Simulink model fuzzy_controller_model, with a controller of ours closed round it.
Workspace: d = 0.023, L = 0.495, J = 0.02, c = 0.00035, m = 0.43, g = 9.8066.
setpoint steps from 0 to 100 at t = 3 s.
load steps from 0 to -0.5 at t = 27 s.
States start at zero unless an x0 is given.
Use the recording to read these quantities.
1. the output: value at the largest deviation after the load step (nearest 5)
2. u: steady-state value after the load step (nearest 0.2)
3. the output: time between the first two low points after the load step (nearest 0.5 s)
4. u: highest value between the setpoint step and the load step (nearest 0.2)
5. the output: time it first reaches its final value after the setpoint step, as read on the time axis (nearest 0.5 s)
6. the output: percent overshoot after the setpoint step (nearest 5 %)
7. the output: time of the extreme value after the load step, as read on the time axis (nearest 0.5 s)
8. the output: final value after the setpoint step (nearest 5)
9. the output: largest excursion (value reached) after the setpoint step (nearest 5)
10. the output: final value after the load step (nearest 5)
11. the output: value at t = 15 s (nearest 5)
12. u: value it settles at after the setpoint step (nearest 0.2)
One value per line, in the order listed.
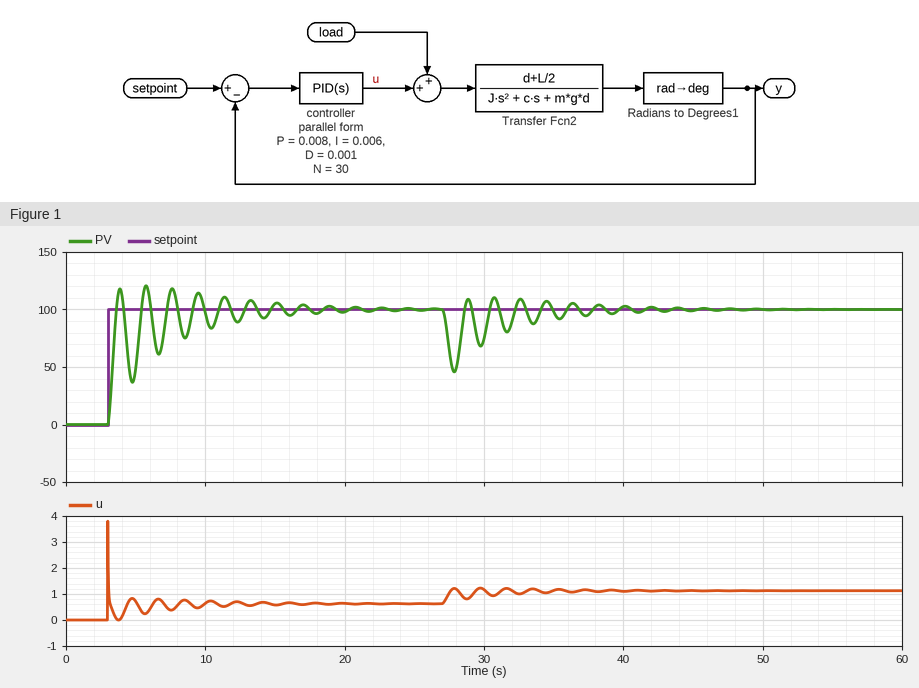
45
1.2
2.0 s
3.8
3.5 s
20 %
28.0 s
100
120
100
105
0.6
